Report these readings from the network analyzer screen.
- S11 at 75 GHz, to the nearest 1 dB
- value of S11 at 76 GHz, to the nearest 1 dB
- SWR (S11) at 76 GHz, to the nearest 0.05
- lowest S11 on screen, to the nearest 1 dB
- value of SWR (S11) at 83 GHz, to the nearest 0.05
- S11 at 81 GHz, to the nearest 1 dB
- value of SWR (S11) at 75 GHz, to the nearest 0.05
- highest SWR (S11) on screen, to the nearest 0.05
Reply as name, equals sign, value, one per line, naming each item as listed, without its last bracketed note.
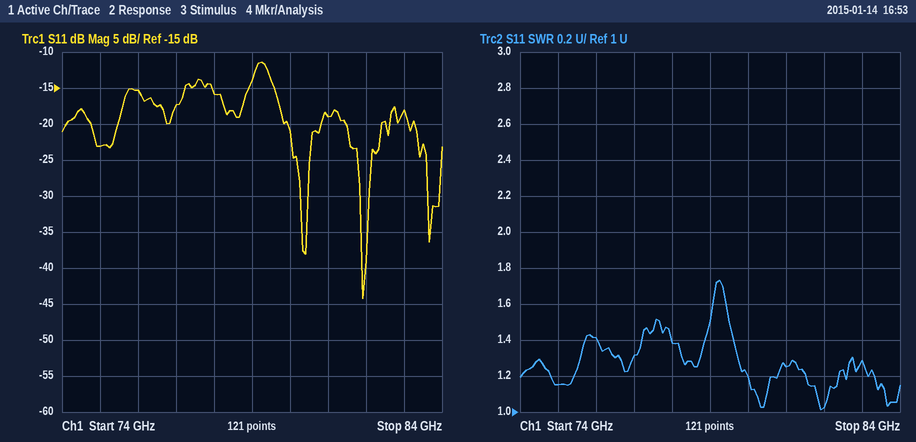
S11 at 75 GHz, to the nearest 1 dB = -23 dB
value of S11 at 76 GHz, to the nearest 1 dB = -15 dB
SWR (S11) at 76 GHz, to the nearest 0.05 = 1.40
lowest S11 on screen, to the nearest 1 dB = -44 dB
value of SWR (S11) at 83 GHz, to the nearest 0.05 = 1.30
S11 at 81 GHz, to the nearest 1 dB = -19 dB
value of SWR (S11) at 75 GHz, to the nearest 0.05 = 1.15
highest SWR (S11) on screen, to the nearest 0.05 = 1.75
